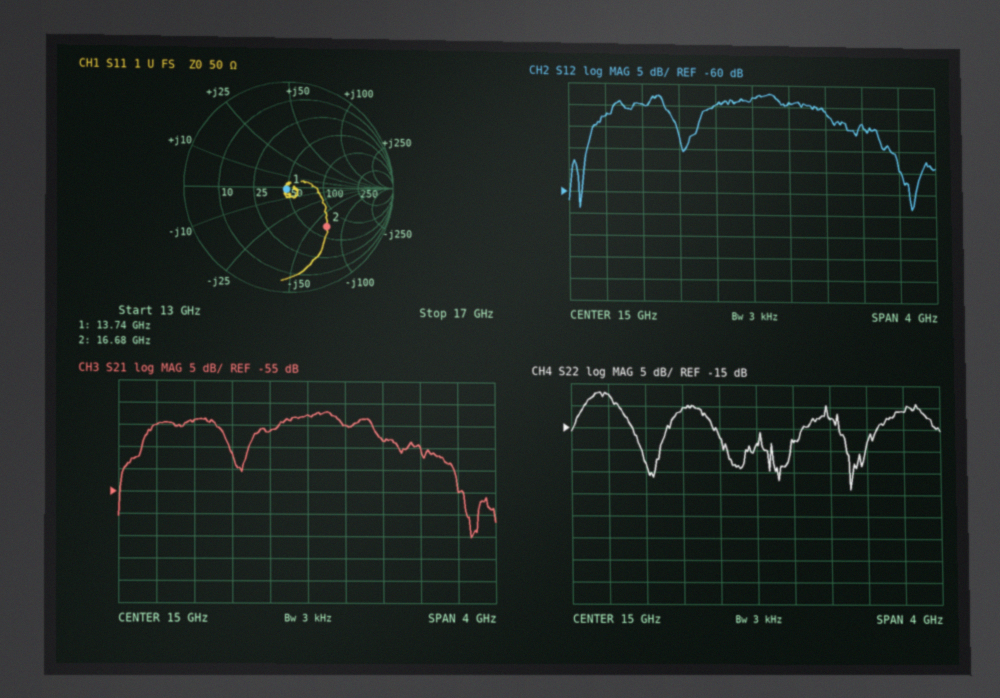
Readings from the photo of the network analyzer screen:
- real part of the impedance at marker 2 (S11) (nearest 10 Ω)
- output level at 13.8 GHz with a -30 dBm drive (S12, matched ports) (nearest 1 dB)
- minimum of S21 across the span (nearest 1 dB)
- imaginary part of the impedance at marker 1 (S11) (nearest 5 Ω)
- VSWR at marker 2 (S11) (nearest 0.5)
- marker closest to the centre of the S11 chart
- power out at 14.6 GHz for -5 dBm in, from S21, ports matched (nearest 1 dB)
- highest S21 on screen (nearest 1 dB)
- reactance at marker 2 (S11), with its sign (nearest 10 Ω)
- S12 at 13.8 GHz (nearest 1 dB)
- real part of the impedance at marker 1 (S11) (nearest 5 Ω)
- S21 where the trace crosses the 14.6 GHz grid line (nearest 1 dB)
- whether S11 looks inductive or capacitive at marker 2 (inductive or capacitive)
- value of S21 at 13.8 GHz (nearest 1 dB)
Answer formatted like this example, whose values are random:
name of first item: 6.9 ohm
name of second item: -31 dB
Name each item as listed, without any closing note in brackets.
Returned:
real part of the impedance at marker 2 (S11): 70 Ω
output level at 13.8 GHz with a -30 dBm drive (S12, matched ports): -70 dBm
minimum of S21 across the span: -65 dB
imaginary part of the impedance at marker 1 (S11): 0 Ω
VSWR at marker 2 (S11): 3.0
marker closest to the centre of the S11 chart: marker 1
power out at 14.6 GHz for -5 dBm in, from S21, ports matched: -46 dBm
highest S21 on screen: -37 dB
reactance at marker 2 (S11), with its sign: -70 Ω
S12 at 13.8 GHz: -40 dB
real part of the impedance at marker 1 (S11): 50 Ω
S21 where the trace crosses the 14.6 GHz grid line: -41 dB
whether S11 looks inductive or capacitive at marker 2: capacitive
value of S21 at 13.8 GHz: -39 dB
